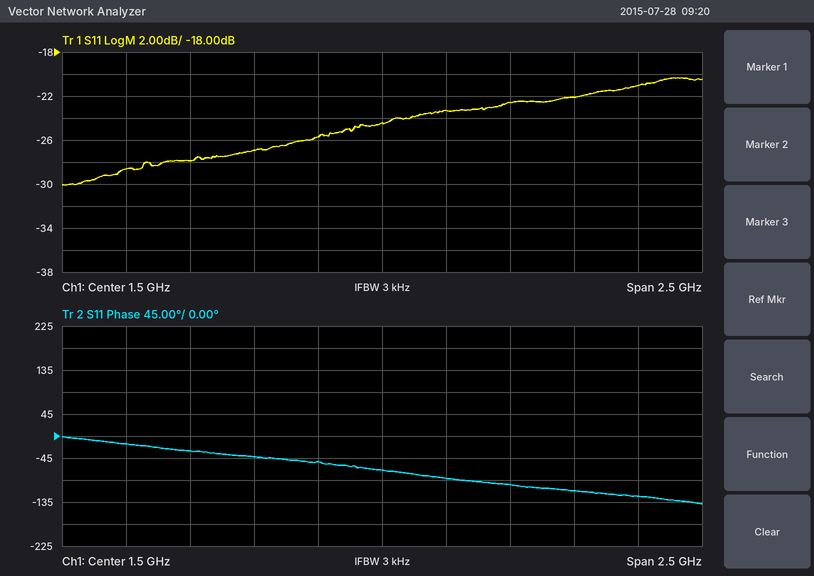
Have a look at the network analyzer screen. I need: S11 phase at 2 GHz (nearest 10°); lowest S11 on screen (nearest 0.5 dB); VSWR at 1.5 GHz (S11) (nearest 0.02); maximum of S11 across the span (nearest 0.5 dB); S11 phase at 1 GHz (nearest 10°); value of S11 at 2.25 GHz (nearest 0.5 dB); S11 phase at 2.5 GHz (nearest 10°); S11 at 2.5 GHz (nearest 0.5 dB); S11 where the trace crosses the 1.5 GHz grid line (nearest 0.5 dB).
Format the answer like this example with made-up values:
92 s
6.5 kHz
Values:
-100°
-30.0 dB
1.12
-20.5 dB
-40°
-22.0 dB
-120°
-21.0 dB
-24.5 dB
